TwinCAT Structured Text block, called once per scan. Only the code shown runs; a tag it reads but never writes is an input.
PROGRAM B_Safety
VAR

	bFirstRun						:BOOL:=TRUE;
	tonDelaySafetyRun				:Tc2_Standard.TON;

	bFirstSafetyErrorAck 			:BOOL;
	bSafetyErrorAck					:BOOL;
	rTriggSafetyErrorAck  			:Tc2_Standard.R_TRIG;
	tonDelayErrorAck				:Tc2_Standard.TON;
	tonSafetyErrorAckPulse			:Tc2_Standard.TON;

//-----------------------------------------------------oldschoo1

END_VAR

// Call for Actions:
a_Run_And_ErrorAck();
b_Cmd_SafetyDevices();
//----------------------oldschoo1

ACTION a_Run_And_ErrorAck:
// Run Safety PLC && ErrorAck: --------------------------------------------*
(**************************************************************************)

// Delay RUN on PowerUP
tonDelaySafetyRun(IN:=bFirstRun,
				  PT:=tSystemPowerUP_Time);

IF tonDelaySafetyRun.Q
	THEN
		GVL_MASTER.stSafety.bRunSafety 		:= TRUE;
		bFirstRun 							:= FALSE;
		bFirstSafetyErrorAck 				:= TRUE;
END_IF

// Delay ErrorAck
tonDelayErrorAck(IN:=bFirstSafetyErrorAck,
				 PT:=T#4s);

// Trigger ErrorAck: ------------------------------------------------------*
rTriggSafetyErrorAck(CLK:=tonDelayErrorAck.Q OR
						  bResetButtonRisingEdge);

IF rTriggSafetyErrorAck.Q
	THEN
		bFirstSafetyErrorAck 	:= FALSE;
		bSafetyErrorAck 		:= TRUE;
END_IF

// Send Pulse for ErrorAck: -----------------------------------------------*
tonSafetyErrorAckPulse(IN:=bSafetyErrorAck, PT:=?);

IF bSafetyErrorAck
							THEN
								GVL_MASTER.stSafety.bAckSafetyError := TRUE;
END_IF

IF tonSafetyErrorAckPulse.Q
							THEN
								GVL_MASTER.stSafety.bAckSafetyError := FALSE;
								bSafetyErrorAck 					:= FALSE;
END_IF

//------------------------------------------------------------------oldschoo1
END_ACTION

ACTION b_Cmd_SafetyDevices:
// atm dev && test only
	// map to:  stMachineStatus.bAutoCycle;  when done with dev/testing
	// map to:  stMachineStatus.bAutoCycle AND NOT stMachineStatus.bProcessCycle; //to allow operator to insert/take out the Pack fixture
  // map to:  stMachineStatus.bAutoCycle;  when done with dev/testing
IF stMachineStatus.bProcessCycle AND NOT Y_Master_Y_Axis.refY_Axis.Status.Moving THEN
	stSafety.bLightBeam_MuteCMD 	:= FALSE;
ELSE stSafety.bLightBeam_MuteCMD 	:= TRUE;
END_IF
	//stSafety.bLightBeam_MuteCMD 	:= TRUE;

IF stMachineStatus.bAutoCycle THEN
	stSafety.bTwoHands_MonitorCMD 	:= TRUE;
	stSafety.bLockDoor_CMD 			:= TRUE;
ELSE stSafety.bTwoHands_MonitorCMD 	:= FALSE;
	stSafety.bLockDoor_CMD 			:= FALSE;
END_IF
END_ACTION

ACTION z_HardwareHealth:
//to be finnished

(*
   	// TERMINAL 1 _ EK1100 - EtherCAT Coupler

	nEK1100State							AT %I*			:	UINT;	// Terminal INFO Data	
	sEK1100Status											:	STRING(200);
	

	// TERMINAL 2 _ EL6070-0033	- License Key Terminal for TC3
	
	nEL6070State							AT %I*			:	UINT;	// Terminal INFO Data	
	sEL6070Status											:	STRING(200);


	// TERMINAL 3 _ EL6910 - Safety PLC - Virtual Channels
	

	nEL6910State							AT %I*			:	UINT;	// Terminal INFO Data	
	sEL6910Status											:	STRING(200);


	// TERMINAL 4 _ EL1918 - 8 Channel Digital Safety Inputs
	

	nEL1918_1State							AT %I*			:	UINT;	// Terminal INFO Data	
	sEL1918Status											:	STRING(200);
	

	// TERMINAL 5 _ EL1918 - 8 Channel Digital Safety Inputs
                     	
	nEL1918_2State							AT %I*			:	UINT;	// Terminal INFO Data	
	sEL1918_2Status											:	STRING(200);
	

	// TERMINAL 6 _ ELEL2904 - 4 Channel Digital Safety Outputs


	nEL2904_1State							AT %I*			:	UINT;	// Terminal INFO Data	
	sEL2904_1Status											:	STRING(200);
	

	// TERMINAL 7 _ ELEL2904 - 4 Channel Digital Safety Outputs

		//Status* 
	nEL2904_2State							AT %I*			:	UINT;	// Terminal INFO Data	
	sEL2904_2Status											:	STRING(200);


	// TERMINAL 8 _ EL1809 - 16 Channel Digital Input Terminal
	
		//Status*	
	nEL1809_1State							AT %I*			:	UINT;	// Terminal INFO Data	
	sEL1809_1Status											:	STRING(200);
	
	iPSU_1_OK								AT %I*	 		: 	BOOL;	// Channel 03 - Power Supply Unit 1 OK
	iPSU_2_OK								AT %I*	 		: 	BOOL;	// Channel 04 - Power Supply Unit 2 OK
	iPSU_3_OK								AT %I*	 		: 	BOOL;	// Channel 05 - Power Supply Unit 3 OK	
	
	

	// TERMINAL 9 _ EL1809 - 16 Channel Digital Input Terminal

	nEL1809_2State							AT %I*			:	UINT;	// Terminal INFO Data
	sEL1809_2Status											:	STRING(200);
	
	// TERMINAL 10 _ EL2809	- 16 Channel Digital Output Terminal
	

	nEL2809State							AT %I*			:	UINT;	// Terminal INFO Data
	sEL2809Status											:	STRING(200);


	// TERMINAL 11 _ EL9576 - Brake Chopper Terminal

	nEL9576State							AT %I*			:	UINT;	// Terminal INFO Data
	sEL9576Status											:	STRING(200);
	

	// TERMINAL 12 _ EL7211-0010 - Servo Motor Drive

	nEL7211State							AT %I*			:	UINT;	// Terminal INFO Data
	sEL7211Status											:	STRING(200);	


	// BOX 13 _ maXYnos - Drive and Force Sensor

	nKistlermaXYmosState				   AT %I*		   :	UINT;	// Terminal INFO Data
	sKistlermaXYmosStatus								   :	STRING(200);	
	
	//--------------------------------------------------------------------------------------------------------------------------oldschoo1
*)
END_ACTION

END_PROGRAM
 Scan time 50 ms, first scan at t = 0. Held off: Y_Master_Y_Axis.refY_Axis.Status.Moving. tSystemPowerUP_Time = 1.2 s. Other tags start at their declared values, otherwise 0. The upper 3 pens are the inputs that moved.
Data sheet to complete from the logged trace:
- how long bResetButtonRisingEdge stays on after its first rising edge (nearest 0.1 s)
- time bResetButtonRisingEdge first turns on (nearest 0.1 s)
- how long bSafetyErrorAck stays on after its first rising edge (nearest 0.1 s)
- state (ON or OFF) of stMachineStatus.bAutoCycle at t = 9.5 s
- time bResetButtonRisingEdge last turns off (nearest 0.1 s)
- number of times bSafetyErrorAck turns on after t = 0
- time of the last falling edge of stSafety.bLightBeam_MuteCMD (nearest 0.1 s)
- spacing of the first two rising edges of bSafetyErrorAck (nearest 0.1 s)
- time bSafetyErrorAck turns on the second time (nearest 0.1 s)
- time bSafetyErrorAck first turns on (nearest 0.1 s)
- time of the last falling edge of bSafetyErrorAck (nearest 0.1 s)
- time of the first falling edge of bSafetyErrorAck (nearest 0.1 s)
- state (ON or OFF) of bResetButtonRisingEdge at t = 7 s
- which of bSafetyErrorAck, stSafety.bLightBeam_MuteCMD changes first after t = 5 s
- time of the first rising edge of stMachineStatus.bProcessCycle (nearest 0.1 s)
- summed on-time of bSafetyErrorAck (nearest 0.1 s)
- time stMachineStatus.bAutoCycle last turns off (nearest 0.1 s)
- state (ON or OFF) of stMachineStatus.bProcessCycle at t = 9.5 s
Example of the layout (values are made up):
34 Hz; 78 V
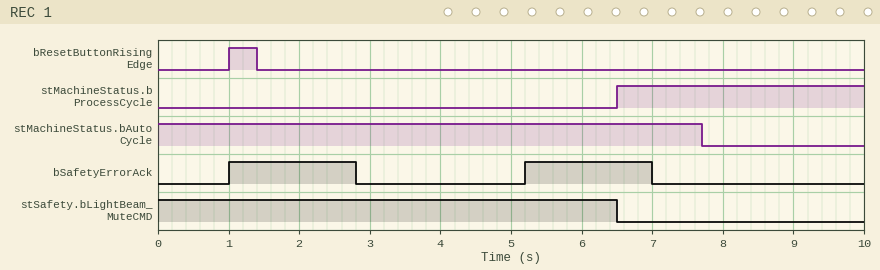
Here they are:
0.4 s; 1.0 s; 1.8 s; OFF; 1.4 s; 2; 6.5 s; 4.2 s; 5.2 s; 1.0 s; 7.0 s; 2.8 s; OFF; bSafetyErrorAck; 6.5 s; 3.6 s; 7.7 s; ON
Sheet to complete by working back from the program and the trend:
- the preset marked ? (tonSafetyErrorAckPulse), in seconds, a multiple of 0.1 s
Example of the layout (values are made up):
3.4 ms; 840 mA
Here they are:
1.8 s
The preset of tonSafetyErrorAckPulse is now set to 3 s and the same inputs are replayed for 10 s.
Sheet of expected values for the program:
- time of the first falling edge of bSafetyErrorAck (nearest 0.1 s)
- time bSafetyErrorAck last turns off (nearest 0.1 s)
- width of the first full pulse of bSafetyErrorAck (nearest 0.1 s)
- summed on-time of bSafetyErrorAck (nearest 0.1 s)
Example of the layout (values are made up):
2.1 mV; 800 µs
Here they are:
4.0 s; 8.2 s; 3.0 s; 6.0 s
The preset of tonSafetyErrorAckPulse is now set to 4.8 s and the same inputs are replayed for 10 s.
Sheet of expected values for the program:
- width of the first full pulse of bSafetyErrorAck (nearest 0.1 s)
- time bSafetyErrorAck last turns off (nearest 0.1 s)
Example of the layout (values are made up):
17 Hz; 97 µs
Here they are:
4.8 s; 5.8 s
